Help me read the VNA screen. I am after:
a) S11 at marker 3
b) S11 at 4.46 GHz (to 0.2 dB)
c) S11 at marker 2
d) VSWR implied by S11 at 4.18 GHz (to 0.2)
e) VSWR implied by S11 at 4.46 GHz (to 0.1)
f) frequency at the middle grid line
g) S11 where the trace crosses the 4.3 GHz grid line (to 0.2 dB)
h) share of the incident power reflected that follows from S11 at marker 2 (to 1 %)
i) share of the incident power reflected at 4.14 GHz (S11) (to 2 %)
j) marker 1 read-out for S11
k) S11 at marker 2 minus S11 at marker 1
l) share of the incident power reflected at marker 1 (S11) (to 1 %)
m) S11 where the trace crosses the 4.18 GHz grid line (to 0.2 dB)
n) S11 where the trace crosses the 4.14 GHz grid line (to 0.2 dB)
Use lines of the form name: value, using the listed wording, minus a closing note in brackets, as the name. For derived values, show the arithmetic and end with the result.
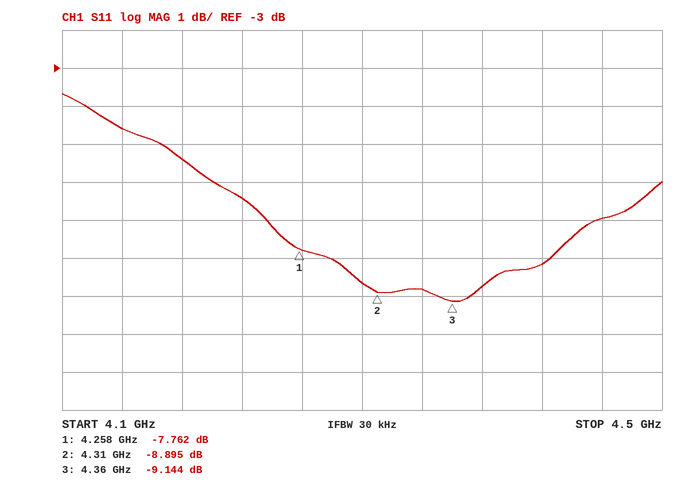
S11 at marker 3: -9.144 dB
S11 at 4.46 GHz: -7.0 dB
S11 at marker 2: -8.895 dB
VSWR implied by S11 at 4.18 GHz: |Γ| = 10^(-5.4/20) = 0.5370; VSWR = (1 + 0.5370)/(1 − 0.5370) ≈ 3.32, so 3.4 to the nearest 0.2
VSWR implied by S11 at 4.46 GHz: |Γ| = 10^(-7/20) = 0.4467; VSWR = (1 + 0.4467)/(1 − 0.4467) ≈ 2.6
frequency at the middle grid line: 4.3 GHz
S11 where the trace crosses the 4.3 GHz grid line: -8.6 dB
share of the incident power reflected that follows from S11 at marker 2: 10^(-8.895/10) ≈ 13 %
share of the incident power reflected at 4.14 GHz (S11): 10^(-4.6/10) ≈ 34.7 %, so 34 % to the nearest 2 %
marker 1 read-out for S11: -7.762 dB
S11 at marker 2 minus S11 at marker 1: -8.895 − (-7.762) = -1.133 dB
share of the incident power reflected at marker 1 (S11): 10^(-7.762/10) ≈ 17 %
S11 where the trace crosses the 4.18 GHz grid line: -5.4 dB
S11 where the trace crosses the 4.14 GHz grid line: -4.6 dB
